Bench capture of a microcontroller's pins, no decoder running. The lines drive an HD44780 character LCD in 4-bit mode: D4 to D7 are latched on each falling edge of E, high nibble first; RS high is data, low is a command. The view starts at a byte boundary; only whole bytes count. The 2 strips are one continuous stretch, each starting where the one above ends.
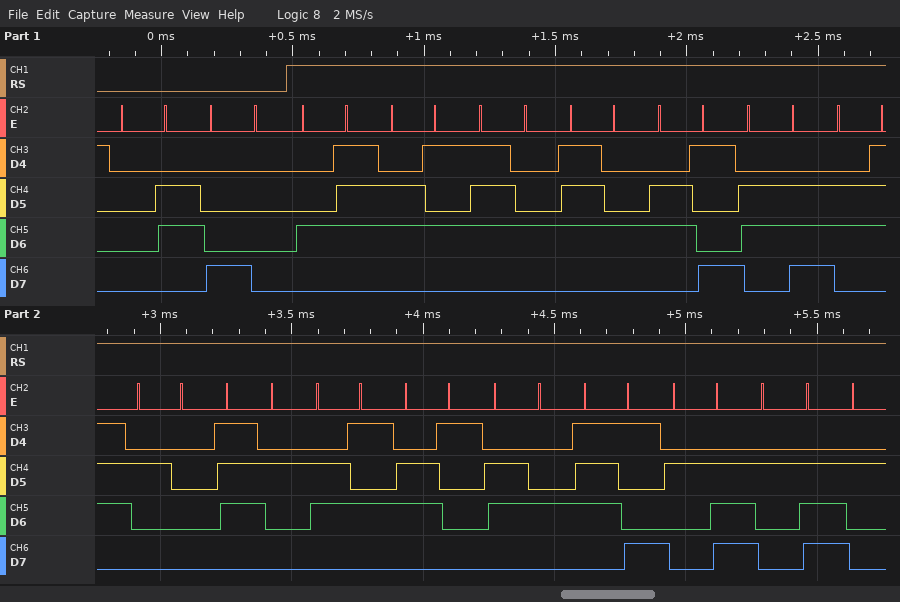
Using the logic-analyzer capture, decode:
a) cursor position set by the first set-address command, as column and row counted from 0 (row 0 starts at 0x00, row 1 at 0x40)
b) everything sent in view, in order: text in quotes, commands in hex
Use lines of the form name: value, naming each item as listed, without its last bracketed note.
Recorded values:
cursor position set by the first set-address command, as column and row counted from 0: column 0, row 0
everything sent in view, in order: text in quotes, commands in hex: 0x06 0x80 "Getting ready.."
